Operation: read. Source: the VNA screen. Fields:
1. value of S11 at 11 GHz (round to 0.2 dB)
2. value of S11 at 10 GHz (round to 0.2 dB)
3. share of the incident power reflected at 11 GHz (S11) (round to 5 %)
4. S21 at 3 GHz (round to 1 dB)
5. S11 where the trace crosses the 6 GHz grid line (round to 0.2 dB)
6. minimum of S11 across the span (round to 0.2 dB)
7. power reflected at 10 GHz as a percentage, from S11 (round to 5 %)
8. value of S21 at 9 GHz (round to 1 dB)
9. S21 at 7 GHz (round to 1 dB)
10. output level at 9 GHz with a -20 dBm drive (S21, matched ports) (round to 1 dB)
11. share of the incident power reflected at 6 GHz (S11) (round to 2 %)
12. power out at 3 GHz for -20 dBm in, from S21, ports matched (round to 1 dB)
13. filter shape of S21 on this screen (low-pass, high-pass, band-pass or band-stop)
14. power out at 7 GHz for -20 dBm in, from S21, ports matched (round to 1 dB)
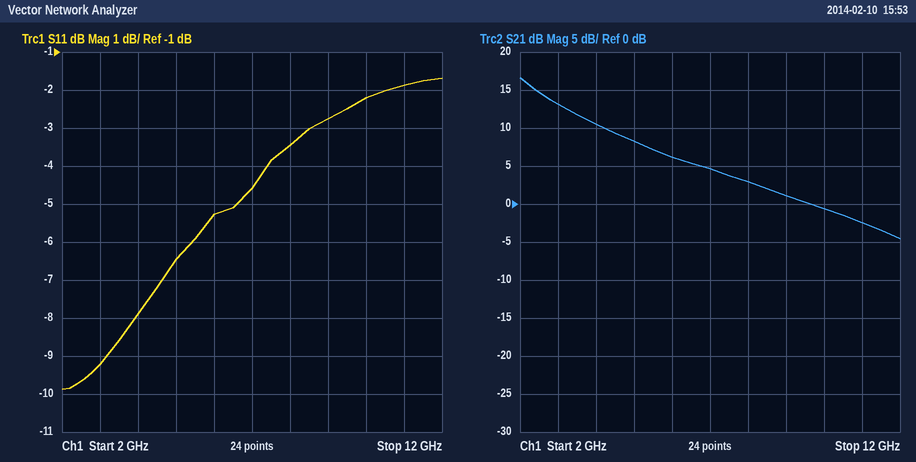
-1.8 dB
-2.2 dB
65 %
13 dB
-5.2 dB
-9.8 dB
60 %
1 dB
5 dB
-19 dBm
30 %
-7 dBm
low-pass
-15 dBm
